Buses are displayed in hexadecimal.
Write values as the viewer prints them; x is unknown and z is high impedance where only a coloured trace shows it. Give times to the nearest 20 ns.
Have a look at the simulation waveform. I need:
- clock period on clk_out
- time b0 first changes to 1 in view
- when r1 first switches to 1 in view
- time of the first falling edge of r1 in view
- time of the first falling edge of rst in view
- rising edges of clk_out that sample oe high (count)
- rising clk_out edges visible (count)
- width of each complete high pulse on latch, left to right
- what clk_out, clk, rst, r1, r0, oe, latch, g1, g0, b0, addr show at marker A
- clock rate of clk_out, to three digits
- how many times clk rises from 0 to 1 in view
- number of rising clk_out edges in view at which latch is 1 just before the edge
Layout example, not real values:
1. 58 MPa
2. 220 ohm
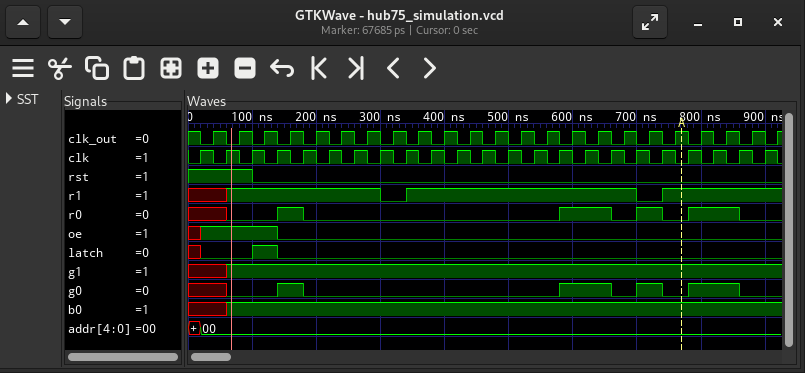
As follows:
1. 40 ns
2. 60 ns
3. 60 ns
4. 300 ns
5. 100 ns
6. 3
7. 23
8. 40 ns
9. clk_out=1, clk=0, rst=0, r1=1, r0=0, oe=0, latch=0, g1=1, g0=0, b0=1, addr=00
10. 25.0 MHz
11. 23
12. 1
